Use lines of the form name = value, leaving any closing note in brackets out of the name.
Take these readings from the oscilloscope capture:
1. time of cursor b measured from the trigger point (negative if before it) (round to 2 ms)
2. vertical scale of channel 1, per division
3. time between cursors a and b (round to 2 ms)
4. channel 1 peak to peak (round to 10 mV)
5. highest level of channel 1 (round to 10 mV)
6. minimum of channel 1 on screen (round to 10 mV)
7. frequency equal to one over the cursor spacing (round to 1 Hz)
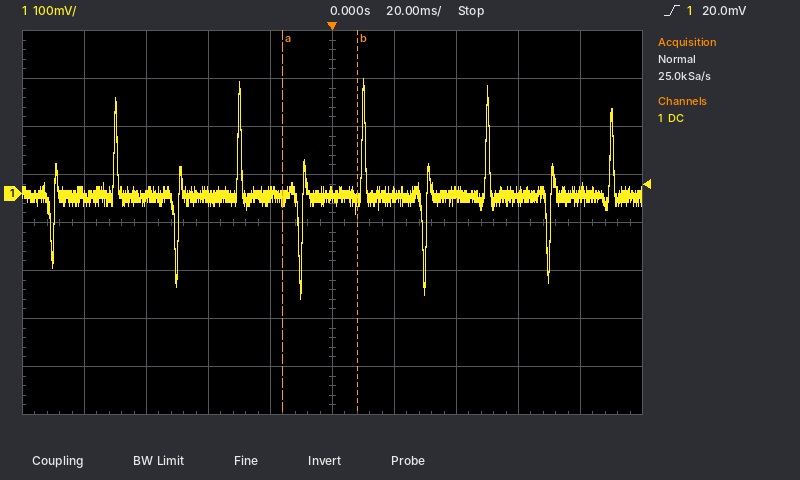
time of cursor b measured from the trigger point (negative if before it) = +8 ms
vertical scale of channel 1, per division = 100 mV
time between cursors a and b = 24 ms
channel 1 peak to peak = 460 mV
highest level of channel 1 = 240 mV
minimum of channel 1 on screen = -220 mV
frequency equal to one over the cursor spacing = 42 Hz
